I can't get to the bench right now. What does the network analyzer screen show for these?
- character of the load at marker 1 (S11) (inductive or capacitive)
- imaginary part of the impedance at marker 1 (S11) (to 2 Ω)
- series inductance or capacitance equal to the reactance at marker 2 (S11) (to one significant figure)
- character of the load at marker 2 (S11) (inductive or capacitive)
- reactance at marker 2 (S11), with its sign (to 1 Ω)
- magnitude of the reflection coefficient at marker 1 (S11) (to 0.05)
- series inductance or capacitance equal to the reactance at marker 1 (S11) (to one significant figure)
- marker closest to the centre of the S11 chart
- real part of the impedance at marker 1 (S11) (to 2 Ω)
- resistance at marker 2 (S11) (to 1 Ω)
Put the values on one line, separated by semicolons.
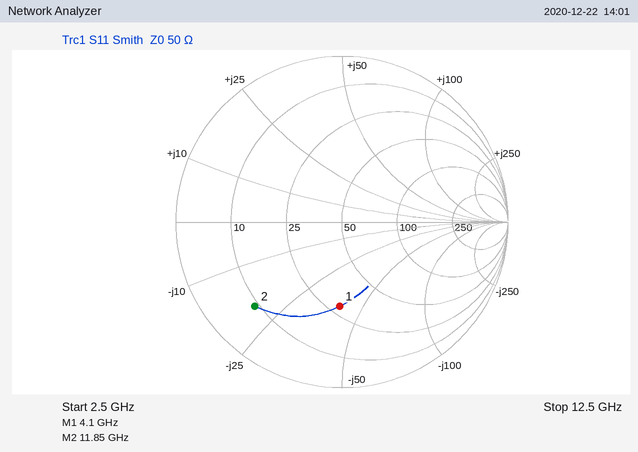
capacitive; -40 Ω; 700 fF; capacitive; -20 Ω; 0.50; 1.0 pF; marker 1; 28 Ω; 9 Ω
